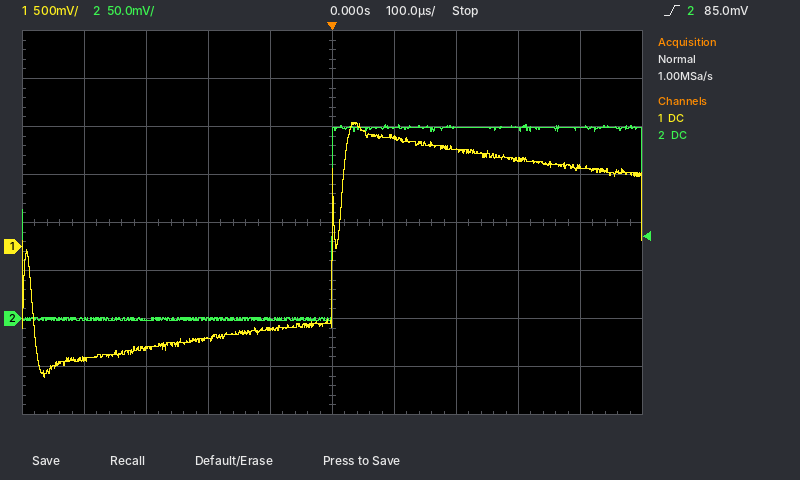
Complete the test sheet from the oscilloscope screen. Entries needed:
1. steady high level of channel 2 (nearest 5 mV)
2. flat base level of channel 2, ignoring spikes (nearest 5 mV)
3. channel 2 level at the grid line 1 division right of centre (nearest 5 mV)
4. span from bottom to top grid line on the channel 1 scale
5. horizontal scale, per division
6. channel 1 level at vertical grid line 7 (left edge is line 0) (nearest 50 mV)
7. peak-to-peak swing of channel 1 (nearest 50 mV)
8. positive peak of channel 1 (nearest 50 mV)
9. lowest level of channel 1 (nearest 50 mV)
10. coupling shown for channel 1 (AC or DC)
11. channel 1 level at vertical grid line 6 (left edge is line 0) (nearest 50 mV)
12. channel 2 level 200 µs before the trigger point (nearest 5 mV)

200 mV
0 mV
200 mV
4 V
100 µs
1.00 V
2.65 V
1.30 V
-1.35 V
DC
1.15 V
0 mV
